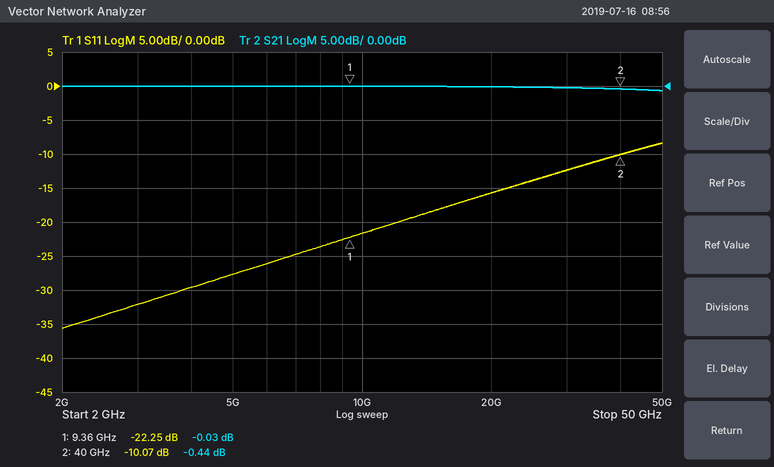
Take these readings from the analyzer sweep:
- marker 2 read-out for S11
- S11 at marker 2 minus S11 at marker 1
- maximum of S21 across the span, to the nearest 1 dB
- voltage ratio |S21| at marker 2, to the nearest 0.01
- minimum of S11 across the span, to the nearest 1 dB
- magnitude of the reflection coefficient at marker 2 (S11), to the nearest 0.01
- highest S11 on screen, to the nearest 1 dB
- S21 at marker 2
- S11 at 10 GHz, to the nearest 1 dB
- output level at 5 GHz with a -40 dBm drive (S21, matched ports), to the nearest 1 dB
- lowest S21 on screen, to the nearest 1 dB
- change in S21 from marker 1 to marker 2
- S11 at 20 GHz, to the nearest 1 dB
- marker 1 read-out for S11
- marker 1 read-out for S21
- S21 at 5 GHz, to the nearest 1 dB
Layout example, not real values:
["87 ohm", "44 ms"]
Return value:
["-10.07 dB", "12.18 dB", "0 dB", "0.95", "-36 dB", "0.31", "-8 dB", "-0.44 dB", "-22 dB", "-40 dBm", "-1 dB", "-0.41 dB", "-16 dB", "-22.25 dB", "-0.03 dB", "0 dB"]
